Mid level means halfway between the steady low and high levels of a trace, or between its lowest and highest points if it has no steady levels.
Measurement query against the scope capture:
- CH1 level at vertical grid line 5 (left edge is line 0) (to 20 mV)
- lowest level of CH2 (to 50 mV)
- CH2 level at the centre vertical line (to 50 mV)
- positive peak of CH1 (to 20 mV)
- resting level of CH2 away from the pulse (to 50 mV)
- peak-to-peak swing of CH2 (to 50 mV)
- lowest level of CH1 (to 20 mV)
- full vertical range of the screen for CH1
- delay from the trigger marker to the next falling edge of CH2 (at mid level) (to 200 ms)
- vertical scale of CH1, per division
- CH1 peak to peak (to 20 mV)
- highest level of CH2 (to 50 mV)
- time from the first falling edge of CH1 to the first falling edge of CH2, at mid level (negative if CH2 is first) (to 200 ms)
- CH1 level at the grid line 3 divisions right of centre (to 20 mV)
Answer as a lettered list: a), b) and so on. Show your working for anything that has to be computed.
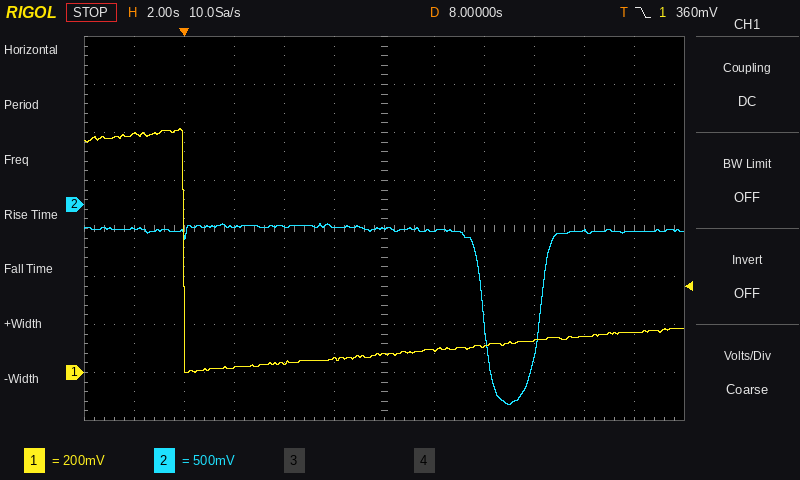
a) 60 mV
b) -2.10 V
c) -250 mV
d) 1.02 V
e) -250 mV
f) -200 mV − (-2.10 V) = 1.90 V
g) 0 mV
h) 1.6 V
i) 12.0 s
j) 200 mV
k) 1.02 V − (0 mV) = 1.02 V
l) -200 mV
m) +12.0 s
n) 140 mV
